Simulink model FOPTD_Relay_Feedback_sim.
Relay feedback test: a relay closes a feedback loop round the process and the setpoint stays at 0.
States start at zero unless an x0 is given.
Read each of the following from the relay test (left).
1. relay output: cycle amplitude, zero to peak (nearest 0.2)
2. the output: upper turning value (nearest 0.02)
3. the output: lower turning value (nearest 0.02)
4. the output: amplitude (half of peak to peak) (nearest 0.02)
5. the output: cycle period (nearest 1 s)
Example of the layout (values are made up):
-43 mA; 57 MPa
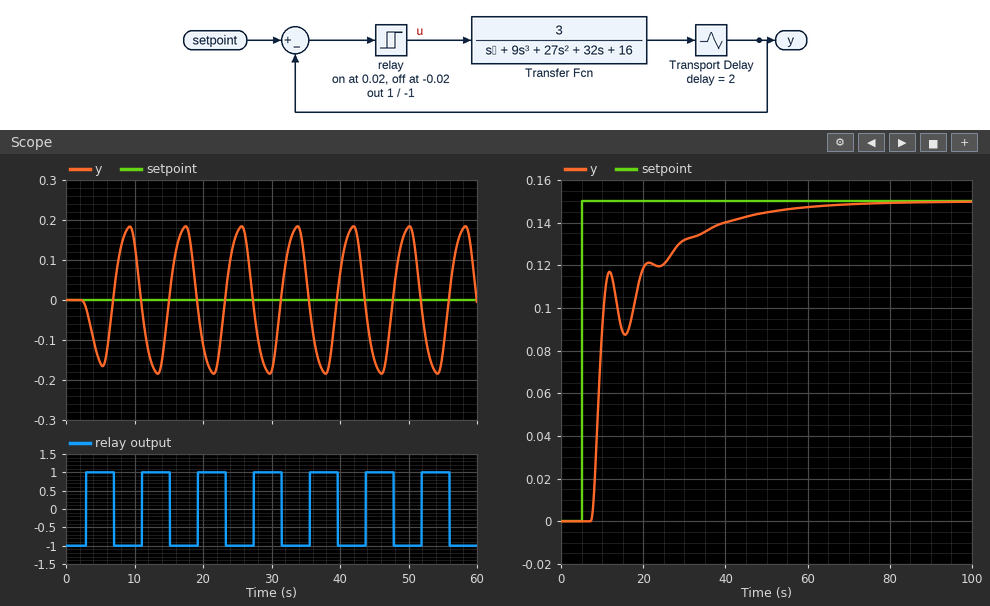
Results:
1.0; 0.18; -0.18; 0.18; 8 s
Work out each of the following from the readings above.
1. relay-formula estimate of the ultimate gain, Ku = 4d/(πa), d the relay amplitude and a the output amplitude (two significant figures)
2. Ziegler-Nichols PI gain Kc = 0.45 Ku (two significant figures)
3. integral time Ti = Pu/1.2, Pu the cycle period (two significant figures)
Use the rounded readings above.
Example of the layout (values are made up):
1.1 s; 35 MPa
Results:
7.1; 3.2; 6.7 s
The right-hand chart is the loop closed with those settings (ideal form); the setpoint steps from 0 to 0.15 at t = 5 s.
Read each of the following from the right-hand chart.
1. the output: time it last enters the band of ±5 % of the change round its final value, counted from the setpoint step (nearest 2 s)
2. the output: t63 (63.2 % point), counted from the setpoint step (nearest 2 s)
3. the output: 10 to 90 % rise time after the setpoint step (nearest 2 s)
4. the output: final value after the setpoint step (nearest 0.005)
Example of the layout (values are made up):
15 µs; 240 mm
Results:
40 s; 6 s; 26 s; 0.150
